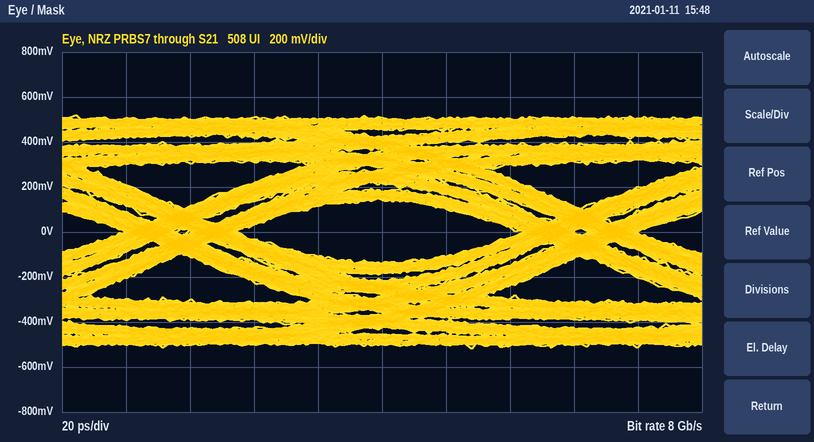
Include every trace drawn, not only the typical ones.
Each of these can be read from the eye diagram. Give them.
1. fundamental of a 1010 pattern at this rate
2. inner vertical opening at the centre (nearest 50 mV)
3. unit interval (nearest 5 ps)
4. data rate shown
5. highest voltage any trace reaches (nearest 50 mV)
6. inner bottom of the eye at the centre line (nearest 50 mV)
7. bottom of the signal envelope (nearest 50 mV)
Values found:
4 GHz
300 mV
125 ps
8 Gb/s
500 mV
-150 mV
-500 mV
